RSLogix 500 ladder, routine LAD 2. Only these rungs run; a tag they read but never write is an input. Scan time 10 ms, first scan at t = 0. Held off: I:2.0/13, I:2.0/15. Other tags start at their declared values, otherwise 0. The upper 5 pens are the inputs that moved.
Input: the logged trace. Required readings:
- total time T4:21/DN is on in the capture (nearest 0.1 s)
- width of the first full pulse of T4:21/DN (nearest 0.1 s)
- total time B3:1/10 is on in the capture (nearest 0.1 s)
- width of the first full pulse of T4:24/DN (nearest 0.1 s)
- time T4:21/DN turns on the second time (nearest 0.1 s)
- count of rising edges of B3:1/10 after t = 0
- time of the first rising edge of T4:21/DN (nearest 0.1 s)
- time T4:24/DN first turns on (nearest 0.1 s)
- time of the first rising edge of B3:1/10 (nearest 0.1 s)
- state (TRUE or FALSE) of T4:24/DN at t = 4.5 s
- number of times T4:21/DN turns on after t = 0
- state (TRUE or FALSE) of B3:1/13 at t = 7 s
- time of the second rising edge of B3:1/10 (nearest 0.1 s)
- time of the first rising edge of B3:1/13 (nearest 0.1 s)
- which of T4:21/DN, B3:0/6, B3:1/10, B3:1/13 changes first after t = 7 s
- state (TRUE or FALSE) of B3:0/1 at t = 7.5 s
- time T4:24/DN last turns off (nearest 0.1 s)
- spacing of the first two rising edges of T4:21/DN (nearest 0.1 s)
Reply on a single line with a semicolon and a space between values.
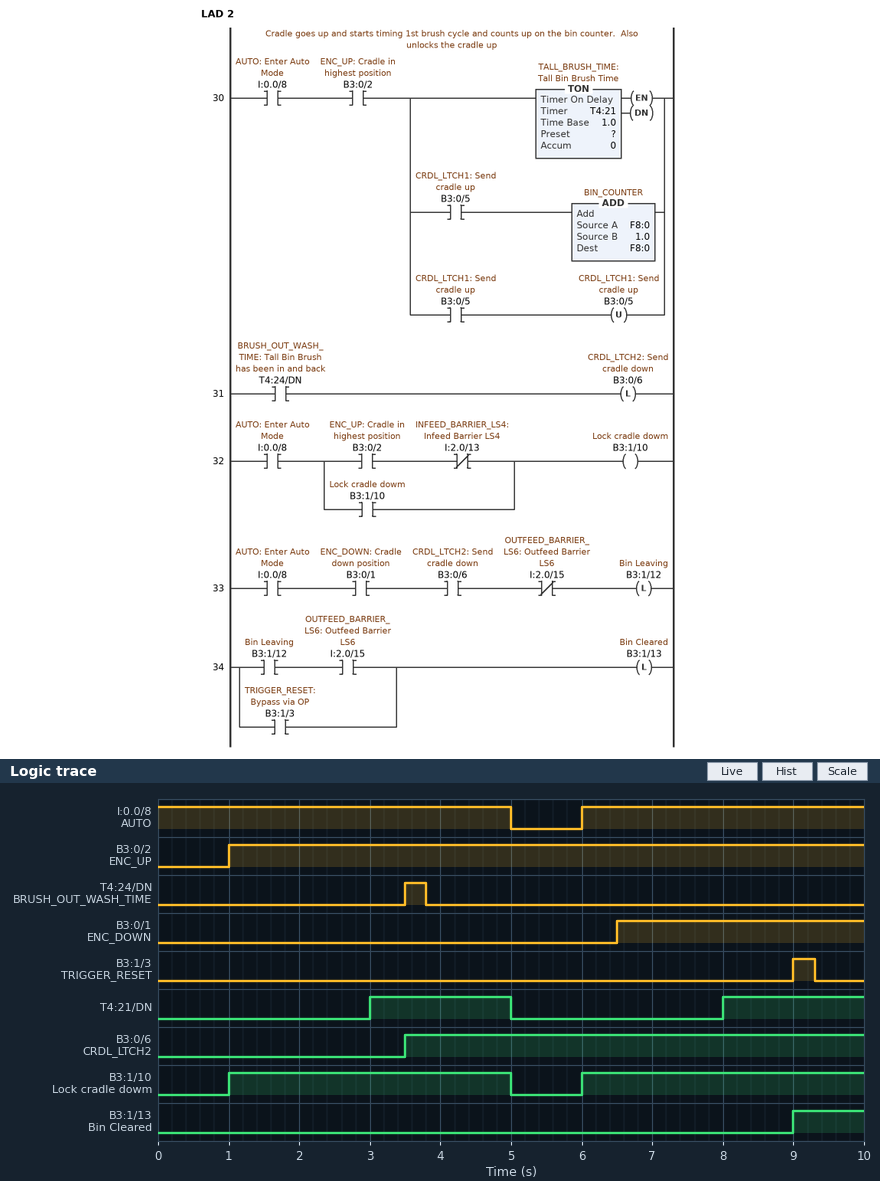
4.0 s; 2.0 s; 8.0 s; 0.3 s; 8.0 s; 2; 3.0 s; 3.5 s; 1.0 s; FALSE; 2; FALSE; 6.0 s; 9.0 s; T4:21/DN; TRUE; 3.8 s; 5.0 s
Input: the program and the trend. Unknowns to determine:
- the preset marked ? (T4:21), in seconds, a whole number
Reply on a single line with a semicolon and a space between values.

2 s
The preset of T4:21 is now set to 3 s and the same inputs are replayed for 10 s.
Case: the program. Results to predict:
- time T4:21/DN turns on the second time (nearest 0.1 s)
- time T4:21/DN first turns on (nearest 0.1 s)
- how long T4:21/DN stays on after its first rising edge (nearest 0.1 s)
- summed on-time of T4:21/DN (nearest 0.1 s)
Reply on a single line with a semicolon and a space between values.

9.0 s; 4.0 s; 1.0 s; 2.0 s
